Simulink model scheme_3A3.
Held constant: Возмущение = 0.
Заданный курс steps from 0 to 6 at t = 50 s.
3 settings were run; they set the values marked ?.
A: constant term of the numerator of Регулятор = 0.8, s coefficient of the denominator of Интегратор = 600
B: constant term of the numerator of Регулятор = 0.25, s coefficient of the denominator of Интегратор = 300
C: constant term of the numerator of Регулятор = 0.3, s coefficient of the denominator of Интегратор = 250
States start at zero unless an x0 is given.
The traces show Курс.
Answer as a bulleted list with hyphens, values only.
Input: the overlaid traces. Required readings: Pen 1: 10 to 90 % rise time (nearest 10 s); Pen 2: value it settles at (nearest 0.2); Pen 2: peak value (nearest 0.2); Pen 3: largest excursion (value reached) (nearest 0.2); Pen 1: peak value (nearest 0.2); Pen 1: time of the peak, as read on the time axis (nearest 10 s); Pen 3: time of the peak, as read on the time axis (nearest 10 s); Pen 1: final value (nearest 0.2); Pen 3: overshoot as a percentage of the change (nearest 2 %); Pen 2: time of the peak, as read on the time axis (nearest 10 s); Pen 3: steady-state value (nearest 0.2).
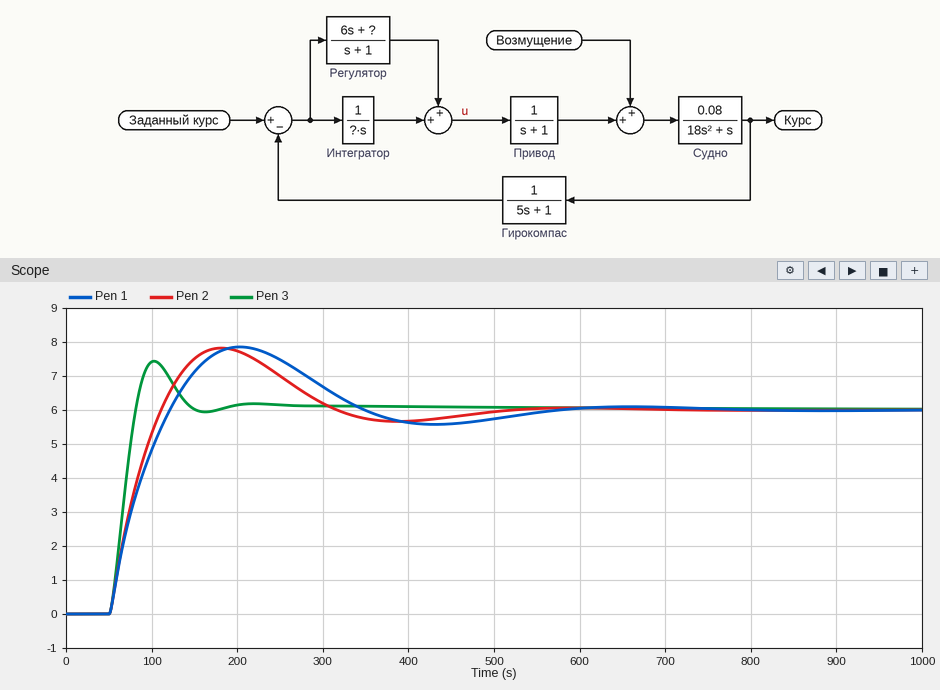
- 50 s
- 6.0
- 7.8
- 7.4
- 7.8
- 200 s
- 100 s
- 6.0
- 24 %
- 180 s
- 6.0
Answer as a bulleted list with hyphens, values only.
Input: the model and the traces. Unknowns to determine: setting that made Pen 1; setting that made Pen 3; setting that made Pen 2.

- B
- A
- C
